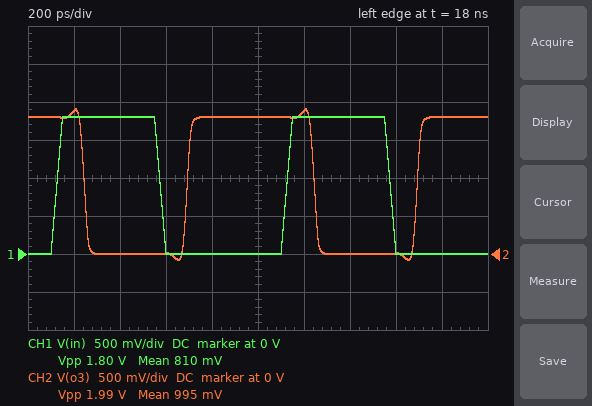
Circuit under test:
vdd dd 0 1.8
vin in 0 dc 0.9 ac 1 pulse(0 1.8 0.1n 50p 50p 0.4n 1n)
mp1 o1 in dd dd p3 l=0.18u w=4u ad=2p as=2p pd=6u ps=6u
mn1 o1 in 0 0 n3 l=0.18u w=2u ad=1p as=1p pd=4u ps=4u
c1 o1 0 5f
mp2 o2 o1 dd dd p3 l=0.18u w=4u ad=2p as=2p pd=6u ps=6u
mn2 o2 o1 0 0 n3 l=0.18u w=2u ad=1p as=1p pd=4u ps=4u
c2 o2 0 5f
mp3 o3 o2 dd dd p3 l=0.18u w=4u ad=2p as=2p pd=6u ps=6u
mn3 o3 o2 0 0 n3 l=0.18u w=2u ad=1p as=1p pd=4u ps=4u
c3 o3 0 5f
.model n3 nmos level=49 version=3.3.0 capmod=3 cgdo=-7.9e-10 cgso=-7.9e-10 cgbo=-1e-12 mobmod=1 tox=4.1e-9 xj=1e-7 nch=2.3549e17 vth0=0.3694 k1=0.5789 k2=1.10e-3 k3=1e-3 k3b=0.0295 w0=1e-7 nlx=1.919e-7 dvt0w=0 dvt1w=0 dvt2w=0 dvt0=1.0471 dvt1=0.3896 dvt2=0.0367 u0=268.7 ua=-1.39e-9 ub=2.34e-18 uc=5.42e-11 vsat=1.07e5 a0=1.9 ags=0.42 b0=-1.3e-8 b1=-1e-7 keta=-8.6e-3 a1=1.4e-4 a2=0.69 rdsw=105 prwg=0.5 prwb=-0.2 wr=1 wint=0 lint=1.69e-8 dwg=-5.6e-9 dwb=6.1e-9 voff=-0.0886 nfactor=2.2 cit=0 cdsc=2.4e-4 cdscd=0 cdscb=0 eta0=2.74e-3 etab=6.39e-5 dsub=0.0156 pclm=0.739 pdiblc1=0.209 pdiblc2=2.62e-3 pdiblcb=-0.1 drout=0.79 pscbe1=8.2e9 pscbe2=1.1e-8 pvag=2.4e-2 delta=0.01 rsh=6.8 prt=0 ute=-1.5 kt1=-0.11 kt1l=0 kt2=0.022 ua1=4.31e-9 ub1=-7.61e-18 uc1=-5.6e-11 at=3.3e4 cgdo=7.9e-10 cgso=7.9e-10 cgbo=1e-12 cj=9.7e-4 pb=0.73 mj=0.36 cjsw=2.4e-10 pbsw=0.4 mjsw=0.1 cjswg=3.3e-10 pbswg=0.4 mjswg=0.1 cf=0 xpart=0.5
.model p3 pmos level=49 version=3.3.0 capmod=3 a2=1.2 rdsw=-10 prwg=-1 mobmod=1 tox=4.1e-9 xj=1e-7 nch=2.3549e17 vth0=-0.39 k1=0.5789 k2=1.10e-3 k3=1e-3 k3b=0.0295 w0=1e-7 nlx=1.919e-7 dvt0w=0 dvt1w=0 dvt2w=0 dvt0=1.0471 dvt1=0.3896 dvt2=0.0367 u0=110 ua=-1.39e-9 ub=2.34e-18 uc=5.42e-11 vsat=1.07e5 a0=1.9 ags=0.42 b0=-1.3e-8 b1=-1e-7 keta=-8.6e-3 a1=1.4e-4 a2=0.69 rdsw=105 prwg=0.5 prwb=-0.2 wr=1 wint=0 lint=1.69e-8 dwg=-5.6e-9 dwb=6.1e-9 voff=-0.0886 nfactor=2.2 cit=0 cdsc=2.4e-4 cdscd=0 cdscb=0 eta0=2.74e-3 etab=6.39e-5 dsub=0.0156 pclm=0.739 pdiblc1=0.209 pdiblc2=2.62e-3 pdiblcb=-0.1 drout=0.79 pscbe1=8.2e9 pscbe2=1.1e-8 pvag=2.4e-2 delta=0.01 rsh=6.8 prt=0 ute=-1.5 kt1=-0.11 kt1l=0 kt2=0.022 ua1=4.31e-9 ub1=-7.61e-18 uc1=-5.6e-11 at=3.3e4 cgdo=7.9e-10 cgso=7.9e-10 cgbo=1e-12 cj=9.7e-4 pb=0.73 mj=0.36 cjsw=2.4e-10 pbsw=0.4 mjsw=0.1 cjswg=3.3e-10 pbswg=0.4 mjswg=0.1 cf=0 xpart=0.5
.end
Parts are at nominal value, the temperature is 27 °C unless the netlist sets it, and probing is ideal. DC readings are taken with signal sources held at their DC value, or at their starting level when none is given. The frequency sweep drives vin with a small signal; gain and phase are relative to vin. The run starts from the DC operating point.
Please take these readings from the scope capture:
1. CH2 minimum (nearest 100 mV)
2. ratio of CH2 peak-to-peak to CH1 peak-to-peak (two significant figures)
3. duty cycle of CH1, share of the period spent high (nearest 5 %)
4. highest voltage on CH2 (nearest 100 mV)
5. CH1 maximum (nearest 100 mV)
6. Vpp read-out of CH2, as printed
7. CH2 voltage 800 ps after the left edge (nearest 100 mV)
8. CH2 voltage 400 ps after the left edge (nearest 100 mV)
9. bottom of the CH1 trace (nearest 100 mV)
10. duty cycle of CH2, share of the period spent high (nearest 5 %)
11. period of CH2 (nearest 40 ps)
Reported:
-100 mV
1.1
45 %
1.9 V
1.8 V
1.99 V
1.8 V
0 V
0 V
55 %
1.00 ns
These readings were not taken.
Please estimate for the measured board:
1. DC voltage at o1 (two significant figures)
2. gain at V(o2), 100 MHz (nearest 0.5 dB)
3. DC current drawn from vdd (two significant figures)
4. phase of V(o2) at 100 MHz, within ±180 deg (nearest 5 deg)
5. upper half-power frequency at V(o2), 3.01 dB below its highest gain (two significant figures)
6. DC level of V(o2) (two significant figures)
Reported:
610 mV
14.0 dB
200 µA
-20 deg
340 MHz
1.8 V
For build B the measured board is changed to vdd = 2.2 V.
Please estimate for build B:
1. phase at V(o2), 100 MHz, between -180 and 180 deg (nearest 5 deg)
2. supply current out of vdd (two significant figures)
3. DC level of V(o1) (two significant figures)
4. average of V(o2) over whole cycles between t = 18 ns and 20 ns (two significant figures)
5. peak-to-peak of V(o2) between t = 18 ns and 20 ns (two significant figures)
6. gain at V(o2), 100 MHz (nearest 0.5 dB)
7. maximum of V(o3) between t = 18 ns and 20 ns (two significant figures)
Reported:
-90 deg
220 µA
2.1 V
950 mV
2.4 V
-60.5 dB
2.3 V
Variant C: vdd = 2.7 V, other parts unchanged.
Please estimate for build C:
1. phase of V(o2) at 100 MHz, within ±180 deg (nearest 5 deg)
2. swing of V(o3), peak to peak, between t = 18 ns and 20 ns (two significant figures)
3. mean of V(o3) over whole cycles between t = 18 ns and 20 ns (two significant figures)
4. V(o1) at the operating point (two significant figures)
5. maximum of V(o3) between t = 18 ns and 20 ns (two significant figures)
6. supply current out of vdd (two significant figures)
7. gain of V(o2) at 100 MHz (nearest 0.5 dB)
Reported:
-90 deg
2.9 V
1.6 V
2.6 V
2.8 V
240 µA
-66.5 dB
